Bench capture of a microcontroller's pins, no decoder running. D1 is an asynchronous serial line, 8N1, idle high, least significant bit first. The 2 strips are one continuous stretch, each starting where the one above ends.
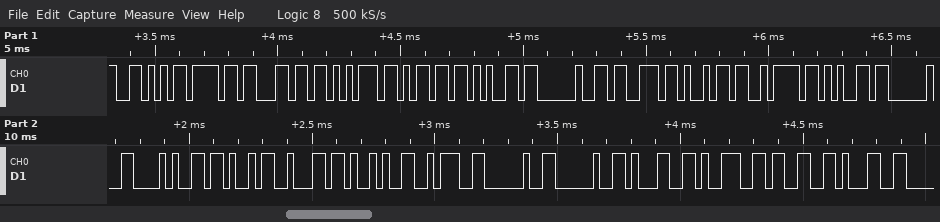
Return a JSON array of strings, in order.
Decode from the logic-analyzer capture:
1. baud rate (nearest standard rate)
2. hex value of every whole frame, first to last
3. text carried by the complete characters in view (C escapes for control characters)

["38400 baud", "56 6F 6C 75 6D 65 20 73 69 7A 65 20 28 4B 62 29 3A 20 20 31 39 33 31", "\"Volume size (Kb):  1931\""]
